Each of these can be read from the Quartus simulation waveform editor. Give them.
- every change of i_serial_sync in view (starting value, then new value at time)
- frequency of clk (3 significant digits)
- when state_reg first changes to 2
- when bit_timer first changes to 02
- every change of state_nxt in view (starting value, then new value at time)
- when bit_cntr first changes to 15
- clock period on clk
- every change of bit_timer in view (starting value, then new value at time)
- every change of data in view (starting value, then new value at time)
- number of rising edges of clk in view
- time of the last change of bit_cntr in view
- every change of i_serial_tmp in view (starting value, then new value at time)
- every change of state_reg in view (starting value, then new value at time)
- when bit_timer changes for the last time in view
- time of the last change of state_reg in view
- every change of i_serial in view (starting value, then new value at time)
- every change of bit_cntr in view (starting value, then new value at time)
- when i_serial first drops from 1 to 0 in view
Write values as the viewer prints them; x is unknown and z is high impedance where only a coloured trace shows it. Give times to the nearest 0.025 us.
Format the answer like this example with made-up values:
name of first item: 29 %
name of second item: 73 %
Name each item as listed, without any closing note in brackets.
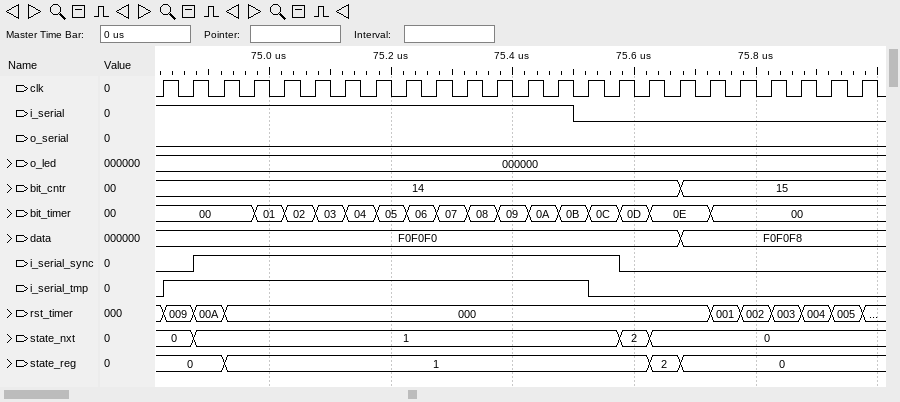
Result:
every change of i_serial_sync in view: 0, 1 at 74.875 us, 0 at 75.575 us
frequency of clk: 20.0 MHz
when state_reg first changes to 2: 75.625 us
when bit_timer first changes to 02: 75.025 us
every change of state_nxt in view: 0, 1 at 74.875 us, 2 at 75.575 us, 0 at 75.625 us
when bit_cntr first changes to 15: 75.675 us
clock period on clk: 0.05 us
every change of bit_timer in view: 00, 01 at 74.975 us, 02 at 75.025 us, 03 at 75.075 us, 04 at 75.125 us, 05 at 75.175 us, 06 at 75.225 us, 07 at 75.275 us, 08 at 75.325 us, 09 at 75.375 us, 0A at 75.425 us, 0B at 75.475 us, 0C at 75.525 us, 0D at 75.575 us, 0E at 75.625 us, 00 at 75.725 us
every change of data in view: F0F0F0, F0F0F8 at 75.675 us
number of rising edges of clk in view: 24
time of the last change of bit_cntr in view: 75.675 us
every change of i_serial_tmp in view: 0, 1 at 74.825 us, 0 at 75.525 us
every change of state_reg in view: 0, 1 at 74.925 us, 2 at 75.625 us, 0 at 75.675 us
when bit_timer changes for the last time in view: 75.725 us
time of the last change of state_reg in view: 75.675 us
every change of i_serial in view: 1, 0 at 75.5 us
every change of bit_cntr in view: 14, 15 at 75.675 us
when i_serial first drops from 1 to 0 in view: 75.5 us
